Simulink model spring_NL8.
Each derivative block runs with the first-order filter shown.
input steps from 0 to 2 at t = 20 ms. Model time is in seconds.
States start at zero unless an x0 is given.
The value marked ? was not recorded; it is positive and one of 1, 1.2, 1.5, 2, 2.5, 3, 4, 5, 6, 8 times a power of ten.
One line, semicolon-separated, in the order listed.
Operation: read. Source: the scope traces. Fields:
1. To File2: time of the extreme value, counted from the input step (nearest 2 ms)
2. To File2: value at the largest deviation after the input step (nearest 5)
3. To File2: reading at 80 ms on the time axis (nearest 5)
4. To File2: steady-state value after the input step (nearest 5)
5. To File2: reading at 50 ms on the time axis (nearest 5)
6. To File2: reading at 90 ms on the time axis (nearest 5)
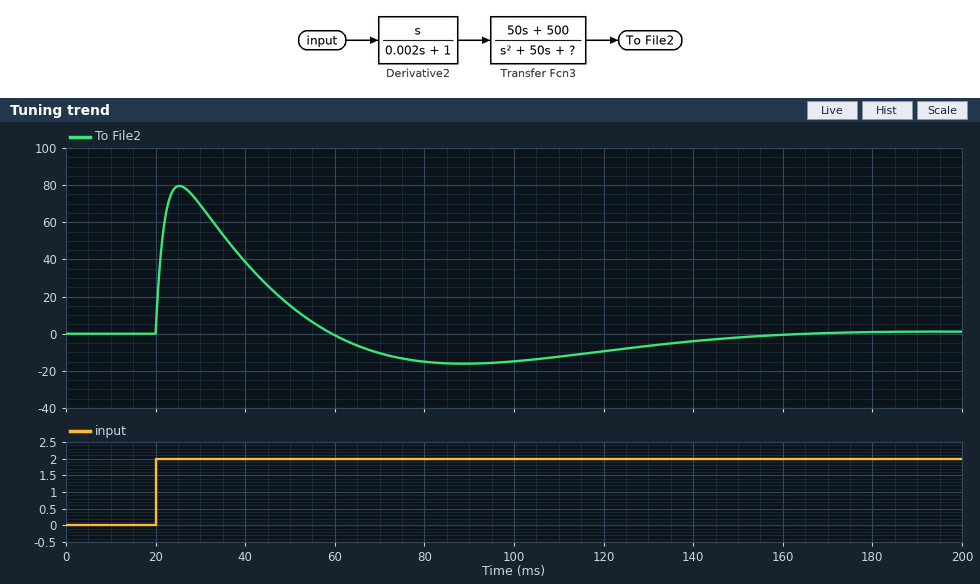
6 ms; 80; -15; 0; 15; -15
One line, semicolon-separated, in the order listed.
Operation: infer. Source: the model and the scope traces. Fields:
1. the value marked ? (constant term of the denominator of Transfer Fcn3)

1500
